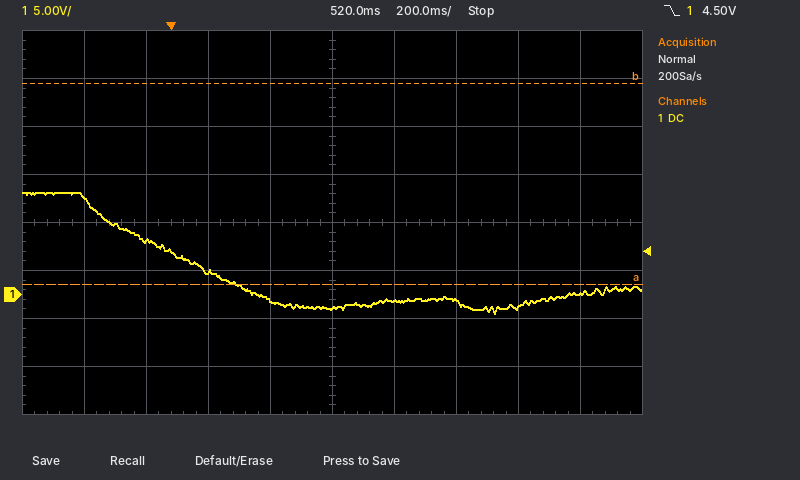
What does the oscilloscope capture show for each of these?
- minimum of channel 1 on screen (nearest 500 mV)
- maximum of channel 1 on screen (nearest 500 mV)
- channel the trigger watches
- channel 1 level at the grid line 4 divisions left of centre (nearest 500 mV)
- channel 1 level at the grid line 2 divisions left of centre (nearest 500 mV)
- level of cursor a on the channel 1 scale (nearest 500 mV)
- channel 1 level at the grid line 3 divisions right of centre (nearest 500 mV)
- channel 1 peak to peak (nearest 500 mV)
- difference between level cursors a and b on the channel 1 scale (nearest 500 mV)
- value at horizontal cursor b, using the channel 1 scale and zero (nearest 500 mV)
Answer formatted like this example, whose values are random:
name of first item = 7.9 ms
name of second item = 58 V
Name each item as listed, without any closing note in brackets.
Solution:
minimum of channel 1 on screen = -2.0 V
maximum of channel 1 on screen = 10.5 V
channel the trigger watches = channel 1
channel 1 level at the grid line 4 divisions left of centre = 10.0 V
channel 1 level at the grid line 2 divisions left of centre = 2.5 V
level of cursor a on the channel 1 scale = 1.0 V
channel 1 level at the grid line 3 divisions right of centre = -1.5 V
channel 1 peak to peak = 12.5 V
difference between level cursors a and b on the channel 1 scale = 21.0 V
value at horizontal cursor b, using the channel 1 scale and zero = 22.0 V
